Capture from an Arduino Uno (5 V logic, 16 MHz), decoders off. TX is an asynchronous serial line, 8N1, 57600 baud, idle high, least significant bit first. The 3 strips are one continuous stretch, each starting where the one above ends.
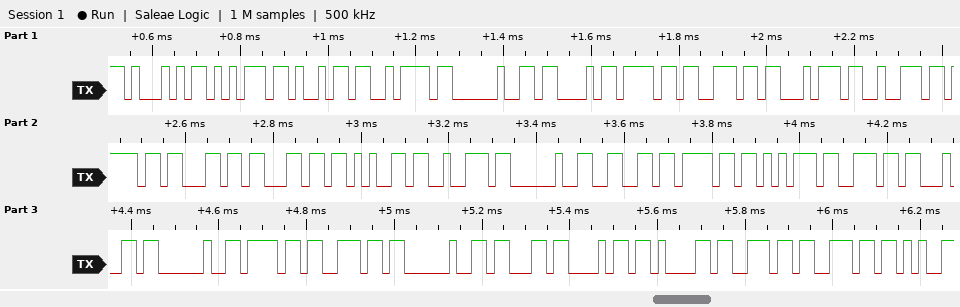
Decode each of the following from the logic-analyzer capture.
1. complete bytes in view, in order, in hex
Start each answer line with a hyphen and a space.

- 51 75 69 7A 20 43 6F 6E 74 72 6F 6C 6C 65 72 20 66 6F 75 6E 64 20 6F 6E 20 63 68 61 6E 6E
